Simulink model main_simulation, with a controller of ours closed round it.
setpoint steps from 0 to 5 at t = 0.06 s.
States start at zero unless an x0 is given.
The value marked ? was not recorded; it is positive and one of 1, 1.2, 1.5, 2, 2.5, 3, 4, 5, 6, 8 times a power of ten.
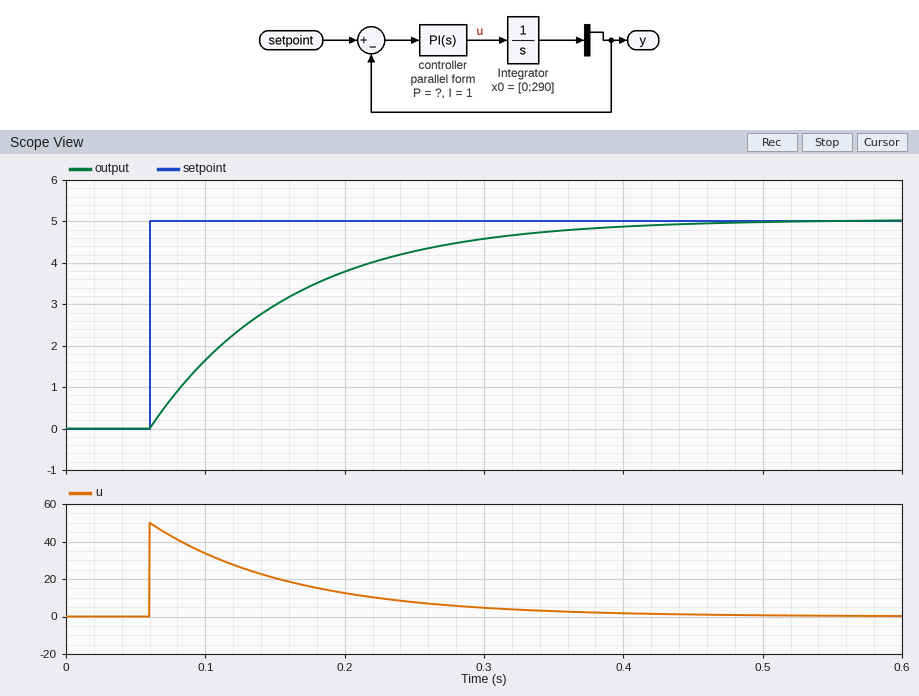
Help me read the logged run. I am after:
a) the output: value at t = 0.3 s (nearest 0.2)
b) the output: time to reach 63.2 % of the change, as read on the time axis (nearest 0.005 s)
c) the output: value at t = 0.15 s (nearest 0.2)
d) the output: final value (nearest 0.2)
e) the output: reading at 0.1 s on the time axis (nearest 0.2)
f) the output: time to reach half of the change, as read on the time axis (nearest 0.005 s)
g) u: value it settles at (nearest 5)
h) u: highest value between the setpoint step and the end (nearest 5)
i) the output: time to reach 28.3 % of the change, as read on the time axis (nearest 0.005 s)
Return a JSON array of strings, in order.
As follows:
["4.6", "0.160 s", "3.0", "5.0", "1.6", "0.130 s", "0", "50", "0.095 s"]
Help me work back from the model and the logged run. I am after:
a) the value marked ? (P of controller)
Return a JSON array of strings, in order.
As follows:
["10"]
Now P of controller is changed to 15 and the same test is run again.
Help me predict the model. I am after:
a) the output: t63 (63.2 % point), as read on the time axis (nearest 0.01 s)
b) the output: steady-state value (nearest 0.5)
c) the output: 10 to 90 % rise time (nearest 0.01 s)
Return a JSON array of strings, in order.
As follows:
["0.13 s", "5.0", "0.15 s"]
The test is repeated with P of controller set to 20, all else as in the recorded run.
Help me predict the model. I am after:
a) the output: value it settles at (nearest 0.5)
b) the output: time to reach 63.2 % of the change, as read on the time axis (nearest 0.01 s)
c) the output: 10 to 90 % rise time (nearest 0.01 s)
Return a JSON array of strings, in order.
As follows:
["5.0", "0.11 s", "0.11 s"]
